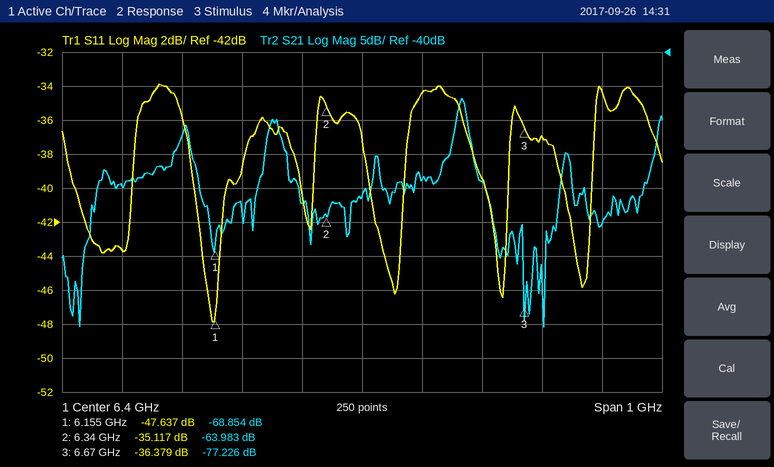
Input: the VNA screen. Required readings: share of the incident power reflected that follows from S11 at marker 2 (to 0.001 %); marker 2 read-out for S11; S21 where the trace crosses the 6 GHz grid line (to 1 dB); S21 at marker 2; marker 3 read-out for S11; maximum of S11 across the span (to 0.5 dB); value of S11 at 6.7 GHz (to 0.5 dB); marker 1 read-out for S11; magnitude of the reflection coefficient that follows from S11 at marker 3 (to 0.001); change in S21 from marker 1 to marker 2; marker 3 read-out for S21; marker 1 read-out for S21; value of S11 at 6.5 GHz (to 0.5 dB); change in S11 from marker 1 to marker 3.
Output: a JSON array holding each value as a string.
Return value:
["0.031 %", "-35.117 dB", "-60 dB", "-63.983 dB", "-36.379 dB", "-34.0 dB", "-37.0 dB", "-47.637 dB", "0.015", "4.871 dB", "-77.226 dB", "-68.854 dB", "-34.5 dB", "11.258 dB"]
